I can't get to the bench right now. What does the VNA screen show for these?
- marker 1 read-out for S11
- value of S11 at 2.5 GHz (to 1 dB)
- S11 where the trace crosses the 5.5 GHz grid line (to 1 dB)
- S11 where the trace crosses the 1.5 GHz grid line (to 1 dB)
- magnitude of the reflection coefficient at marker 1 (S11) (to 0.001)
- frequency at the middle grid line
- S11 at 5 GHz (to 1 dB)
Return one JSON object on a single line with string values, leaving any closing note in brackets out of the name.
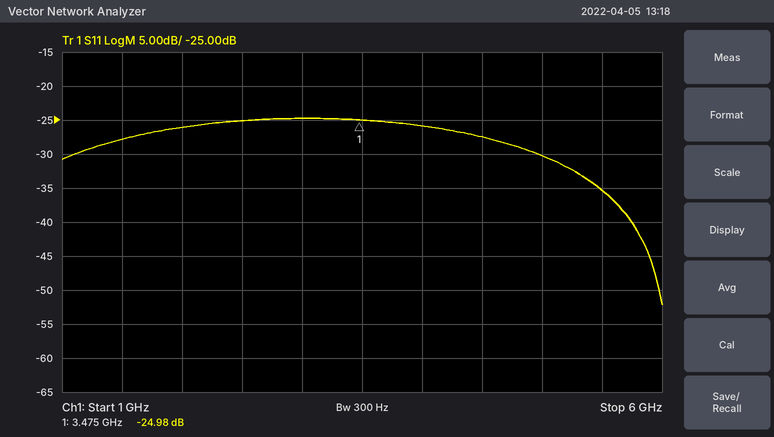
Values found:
{"marker 1 read-out for S11": "-24.98 dB", "value of S11 at 2.5 GHz": "-25 dB", "S11 where the trace crosses the 5.5 GHz grid line": "-35 dB", "S11 where the trace crosses the 1.5 GHz grid line": "-28 dB", "magnitude of the reflection coefficient at marker 1 (S11)": "0.056", "frequency at the middle grid line": "3.5 GHz", "S11 at 5 GHz": "-30 dB"}
